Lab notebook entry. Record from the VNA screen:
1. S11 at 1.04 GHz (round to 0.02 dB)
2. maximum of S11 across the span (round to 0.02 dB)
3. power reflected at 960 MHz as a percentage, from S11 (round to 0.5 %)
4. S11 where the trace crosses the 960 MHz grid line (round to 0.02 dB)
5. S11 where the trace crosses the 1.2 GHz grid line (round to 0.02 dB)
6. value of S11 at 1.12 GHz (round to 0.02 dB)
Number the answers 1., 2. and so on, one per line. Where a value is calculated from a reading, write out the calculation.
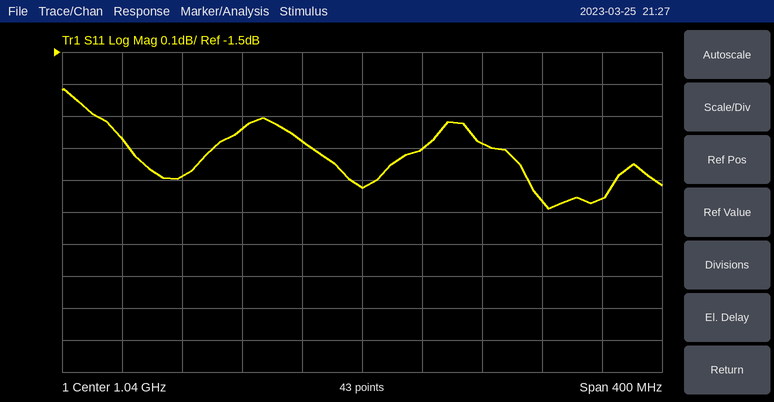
1. -1.92 dB
2. -1.62 dB
3. 10^(-1.74/10) ≈ 67.0 %
4. -1.74 dB
5. -1.96 dB
6. -1.78 dB
